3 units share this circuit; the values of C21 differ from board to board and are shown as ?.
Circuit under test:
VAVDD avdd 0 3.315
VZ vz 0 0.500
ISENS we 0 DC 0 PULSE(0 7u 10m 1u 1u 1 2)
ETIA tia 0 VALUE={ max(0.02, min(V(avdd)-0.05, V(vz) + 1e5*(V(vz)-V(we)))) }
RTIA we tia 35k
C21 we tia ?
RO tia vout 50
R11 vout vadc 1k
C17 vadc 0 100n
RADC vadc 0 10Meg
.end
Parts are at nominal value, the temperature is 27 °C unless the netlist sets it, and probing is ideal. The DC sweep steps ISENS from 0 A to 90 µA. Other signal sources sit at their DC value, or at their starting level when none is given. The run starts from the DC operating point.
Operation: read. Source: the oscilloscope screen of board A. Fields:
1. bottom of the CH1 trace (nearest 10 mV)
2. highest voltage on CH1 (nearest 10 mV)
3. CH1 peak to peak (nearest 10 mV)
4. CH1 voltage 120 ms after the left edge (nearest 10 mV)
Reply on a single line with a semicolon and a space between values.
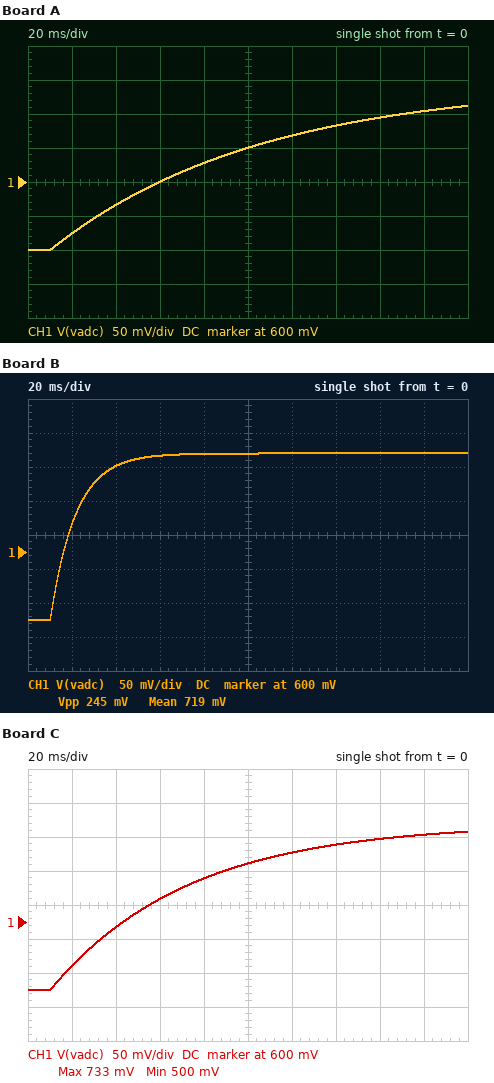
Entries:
500 mV; 710 mV; 210 mV; 670 mV
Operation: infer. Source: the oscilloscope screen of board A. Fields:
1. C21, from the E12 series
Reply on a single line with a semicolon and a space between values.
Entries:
2.7 µF
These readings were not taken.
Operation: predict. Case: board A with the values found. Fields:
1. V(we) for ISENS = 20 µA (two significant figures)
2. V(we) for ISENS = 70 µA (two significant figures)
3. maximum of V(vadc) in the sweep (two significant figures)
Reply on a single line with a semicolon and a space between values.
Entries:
500 mV; 500 mV; 3.3 V
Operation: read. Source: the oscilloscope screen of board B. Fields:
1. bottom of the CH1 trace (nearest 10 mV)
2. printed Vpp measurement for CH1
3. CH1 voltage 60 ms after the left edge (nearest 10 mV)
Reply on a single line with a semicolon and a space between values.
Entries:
500 mV; 245 mV; 740 mV
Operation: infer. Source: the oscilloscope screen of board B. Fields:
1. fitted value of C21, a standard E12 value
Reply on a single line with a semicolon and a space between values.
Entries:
330 nF
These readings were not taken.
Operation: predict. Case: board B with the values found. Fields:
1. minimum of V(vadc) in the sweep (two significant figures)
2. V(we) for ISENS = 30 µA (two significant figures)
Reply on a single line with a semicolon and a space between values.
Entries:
500 mV; 500 mV
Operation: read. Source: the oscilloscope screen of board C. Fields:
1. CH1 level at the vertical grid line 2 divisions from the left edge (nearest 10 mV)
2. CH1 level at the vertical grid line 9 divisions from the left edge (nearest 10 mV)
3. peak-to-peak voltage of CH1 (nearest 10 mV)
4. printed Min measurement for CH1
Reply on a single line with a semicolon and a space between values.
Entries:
590 mV; 730 mV; 230 mV; 500 mV
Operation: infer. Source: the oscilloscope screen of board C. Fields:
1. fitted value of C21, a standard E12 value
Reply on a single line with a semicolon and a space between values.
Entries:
1.8 µF
